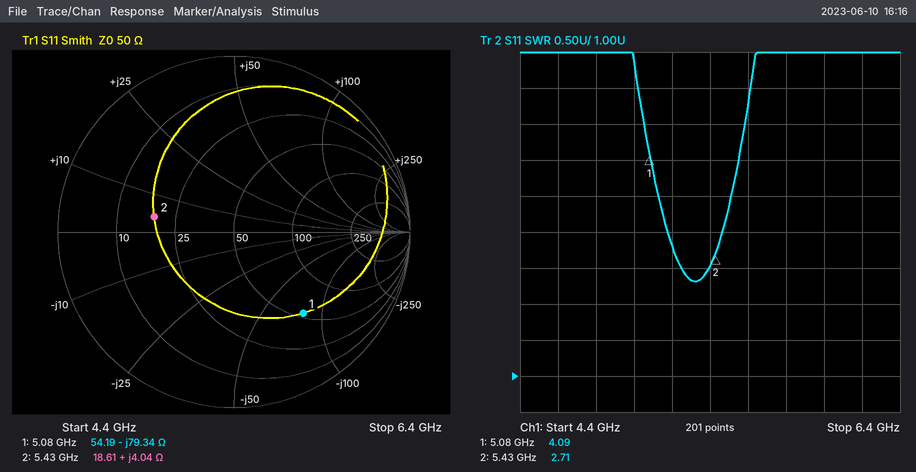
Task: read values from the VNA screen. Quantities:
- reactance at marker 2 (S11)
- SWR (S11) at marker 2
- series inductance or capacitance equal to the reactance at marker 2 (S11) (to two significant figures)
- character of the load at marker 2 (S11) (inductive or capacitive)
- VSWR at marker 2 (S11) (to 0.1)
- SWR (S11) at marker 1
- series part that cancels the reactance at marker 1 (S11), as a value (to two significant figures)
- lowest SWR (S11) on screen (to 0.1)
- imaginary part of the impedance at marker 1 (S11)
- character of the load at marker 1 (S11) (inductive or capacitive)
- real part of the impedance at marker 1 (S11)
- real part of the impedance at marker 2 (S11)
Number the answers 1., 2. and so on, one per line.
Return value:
1. +4.04 Ω
2. 2.71
3. 120 pH
4. inductive
5. 2.7
6. 4.09
7. 2.5 nH
8. 2.3
9. -79.34 Ω
10. capacitive
11. 54.19 Ω
12. 18.61 Ω
